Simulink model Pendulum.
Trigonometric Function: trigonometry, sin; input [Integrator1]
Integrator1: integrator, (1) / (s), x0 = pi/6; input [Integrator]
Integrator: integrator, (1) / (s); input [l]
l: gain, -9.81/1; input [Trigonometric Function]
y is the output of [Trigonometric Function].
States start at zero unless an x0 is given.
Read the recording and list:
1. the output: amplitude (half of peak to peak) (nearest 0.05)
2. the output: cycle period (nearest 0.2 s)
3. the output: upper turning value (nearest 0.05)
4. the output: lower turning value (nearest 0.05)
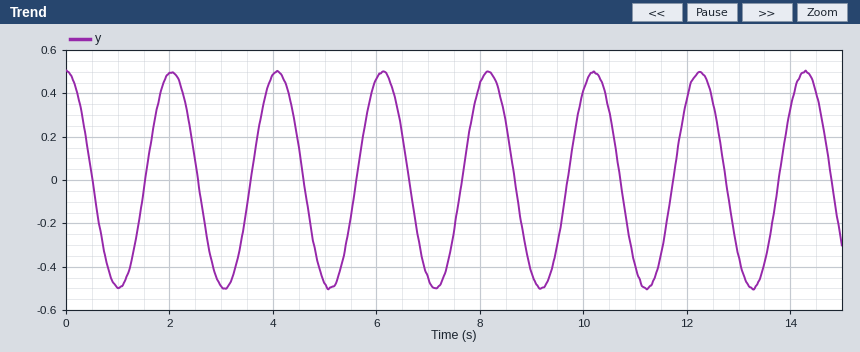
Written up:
0.50
2.0 s
0.50
-0.50
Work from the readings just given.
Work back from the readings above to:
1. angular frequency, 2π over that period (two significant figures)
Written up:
3.1 rad/s
